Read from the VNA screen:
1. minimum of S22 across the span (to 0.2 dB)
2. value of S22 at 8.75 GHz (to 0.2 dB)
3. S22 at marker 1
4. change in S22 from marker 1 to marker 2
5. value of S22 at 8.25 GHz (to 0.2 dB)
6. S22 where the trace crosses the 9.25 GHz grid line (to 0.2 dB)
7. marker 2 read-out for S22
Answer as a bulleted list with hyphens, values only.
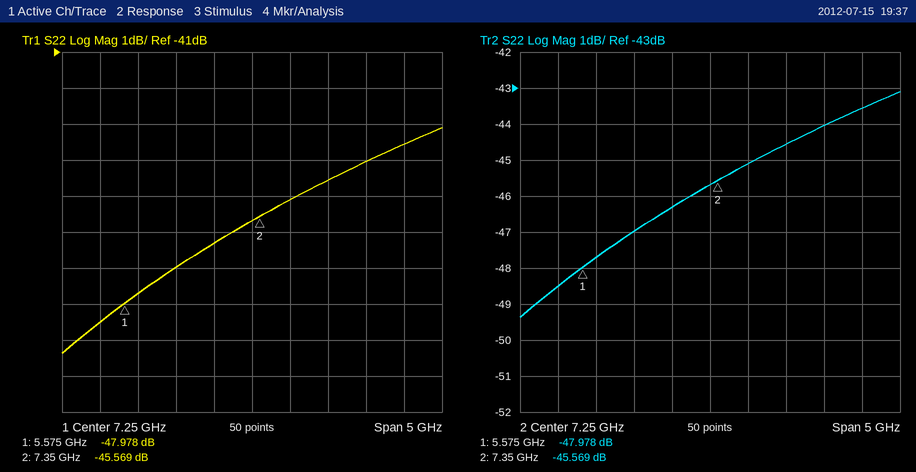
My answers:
- -49.4 dB
- -44.0 dB
- -47.978 dB
- 2.409 dB
- -44.6 dB
- -43.6 dB
- -45.569 dB
